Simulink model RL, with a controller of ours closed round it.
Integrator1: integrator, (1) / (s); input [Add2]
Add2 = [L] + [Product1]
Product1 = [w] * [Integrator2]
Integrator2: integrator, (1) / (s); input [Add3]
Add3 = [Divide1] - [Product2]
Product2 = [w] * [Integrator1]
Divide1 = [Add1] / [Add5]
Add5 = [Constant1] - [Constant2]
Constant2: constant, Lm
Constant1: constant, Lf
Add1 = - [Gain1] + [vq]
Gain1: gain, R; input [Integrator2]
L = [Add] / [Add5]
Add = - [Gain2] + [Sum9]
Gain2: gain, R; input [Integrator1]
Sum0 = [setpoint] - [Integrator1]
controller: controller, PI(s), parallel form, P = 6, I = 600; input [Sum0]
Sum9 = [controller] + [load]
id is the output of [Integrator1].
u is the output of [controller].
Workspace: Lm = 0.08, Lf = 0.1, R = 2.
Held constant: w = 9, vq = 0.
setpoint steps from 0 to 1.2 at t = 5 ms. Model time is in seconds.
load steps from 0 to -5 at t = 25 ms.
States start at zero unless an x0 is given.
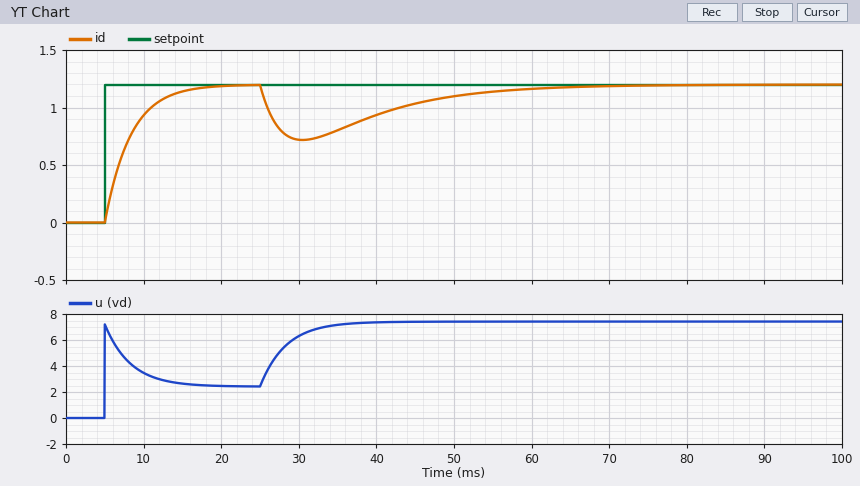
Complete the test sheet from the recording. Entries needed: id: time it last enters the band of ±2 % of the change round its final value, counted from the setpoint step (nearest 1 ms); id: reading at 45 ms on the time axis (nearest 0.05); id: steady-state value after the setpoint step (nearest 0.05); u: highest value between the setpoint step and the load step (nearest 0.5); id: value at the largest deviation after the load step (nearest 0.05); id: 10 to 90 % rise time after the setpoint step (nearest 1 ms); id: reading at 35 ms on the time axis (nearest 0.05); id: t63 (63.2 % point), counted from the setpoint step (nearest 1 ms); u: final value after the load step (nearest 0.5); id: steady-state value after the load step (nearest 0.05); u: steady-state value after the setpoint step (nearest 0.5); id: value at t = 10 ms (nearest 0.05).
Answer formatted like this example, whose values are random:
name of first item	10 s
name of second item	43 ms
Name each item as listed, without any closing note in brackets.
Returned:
id: time it last enters the band of ±2 % of the change round its final value, counted from the setpoint step	13 ms
id: reading at 45 ms on the time axis	1.05
id: steady-state value after the setpoint step	1.20
u: highest value between the setpoint step and the load step	7.0
id: value at the largest deviation after the load step	0.70
id: 10 to 90 % rise time after the setpoint step	7 ms
id: reading at 35 ms on the time axis	0.80
id: t63 (63.2 % point), counted from the setpoint step	3 ms
u: final value after the load step	7.5
id: steady-state value after the load step	1.20
u: steady-state value after the setpoint step	2.5
id: value at t = 10 ms	0.95
